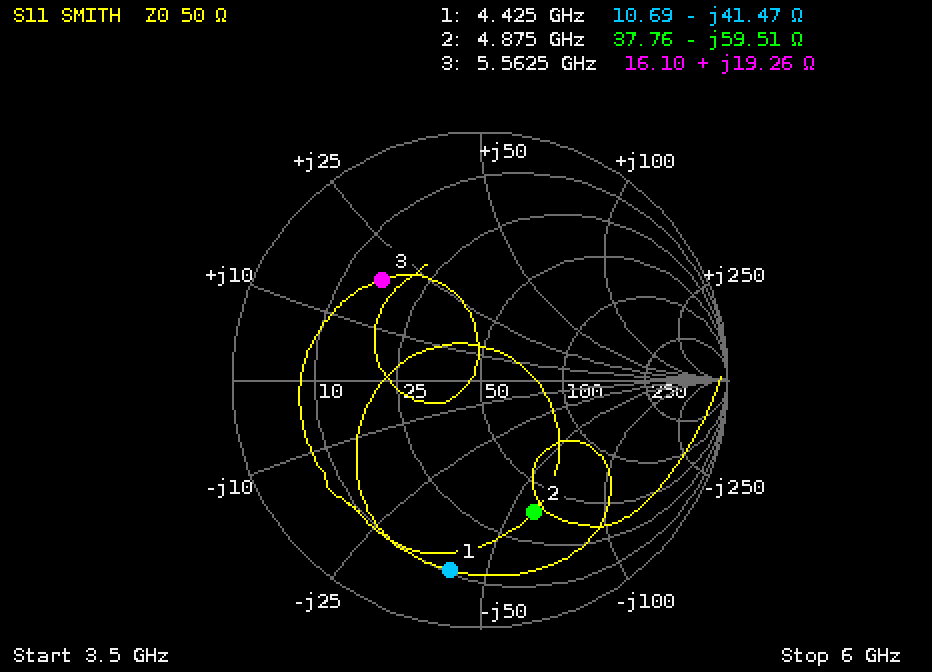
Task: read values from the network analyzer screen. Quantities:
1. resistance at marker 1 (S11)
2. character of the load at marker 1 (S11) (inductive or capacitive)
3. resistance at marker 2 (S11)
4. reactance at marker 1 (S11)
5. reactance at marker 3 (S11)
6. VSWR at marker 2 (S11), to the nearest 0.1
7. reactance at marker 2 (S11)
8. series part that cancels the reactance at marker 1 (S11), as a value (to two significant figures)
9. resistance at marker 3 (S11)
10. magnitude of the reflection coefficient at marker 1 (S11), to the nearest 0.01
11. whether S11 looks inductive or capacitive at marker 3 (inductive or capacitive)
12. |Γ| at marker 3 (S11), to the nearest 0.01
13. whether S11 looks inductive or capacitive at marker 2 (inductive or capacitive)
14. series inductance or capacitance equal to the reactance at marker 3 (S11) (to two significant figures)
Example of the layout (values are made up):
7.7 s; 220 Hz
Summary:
10.69 Ω; capacitive; 37.76 Ω; -41.47 Ω; +19.26 Ω; 3.7; -59.51 Ω; 1.5 nH; 16.10 Ω; 0.78; inductive; 0.57; capacitive; 550 pH
